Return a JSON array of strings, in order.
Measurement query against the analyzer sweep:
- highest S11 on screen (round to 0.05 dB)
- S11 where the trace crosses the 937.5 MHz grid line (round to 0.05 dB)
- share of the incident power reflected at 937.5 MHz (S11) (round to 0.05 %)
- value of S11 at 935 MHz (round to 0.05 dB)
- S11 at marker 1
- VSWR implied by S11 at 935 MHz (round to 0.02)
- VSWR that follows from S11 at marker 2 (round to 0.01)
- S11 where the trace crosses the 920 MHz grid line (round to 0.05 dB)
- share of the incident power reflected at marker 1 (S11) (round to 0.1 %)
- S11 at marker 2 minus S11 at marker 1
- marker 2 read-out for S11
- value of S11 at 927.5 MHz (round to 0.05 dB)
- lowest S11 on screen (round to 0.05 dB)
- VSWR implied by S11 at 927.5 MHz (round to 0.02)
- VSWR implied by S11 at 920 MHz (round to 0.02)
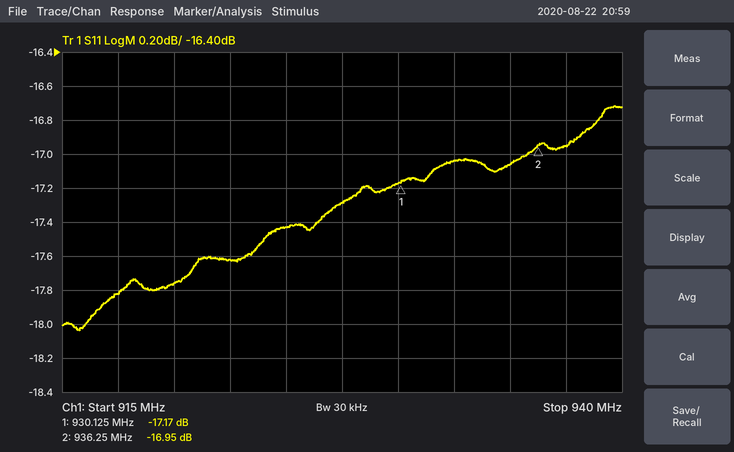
["-16.70 dB", "-16.95 dB", "2.00 %", "-17.05 dB", "-17.17 dB", "1.32", "1.33", "-17.75 dB", "1.9 %", "0.22 dB", "-16.95 dB", "-17.30 dB", "-18.05 dB", "1.32", "1.30"]
